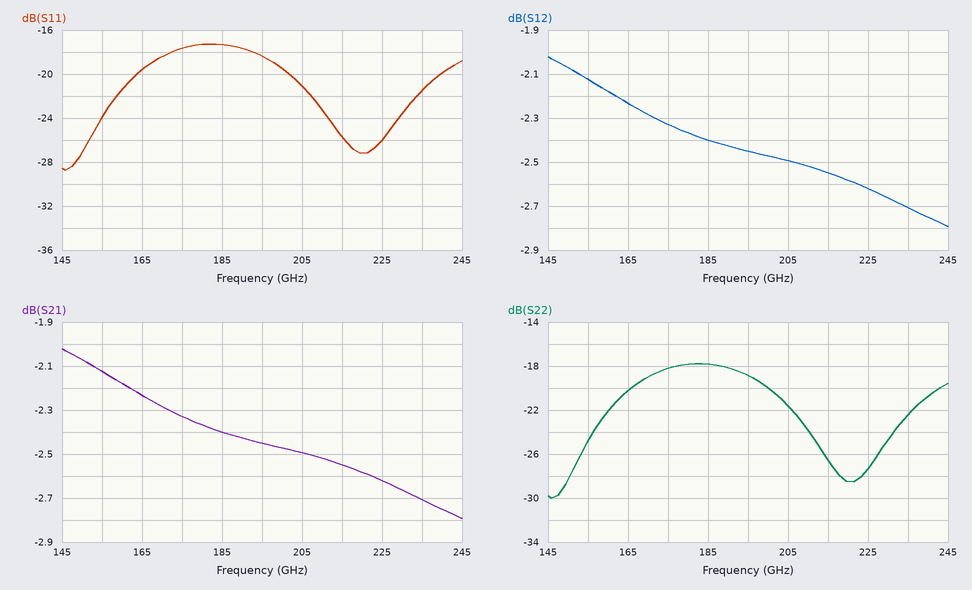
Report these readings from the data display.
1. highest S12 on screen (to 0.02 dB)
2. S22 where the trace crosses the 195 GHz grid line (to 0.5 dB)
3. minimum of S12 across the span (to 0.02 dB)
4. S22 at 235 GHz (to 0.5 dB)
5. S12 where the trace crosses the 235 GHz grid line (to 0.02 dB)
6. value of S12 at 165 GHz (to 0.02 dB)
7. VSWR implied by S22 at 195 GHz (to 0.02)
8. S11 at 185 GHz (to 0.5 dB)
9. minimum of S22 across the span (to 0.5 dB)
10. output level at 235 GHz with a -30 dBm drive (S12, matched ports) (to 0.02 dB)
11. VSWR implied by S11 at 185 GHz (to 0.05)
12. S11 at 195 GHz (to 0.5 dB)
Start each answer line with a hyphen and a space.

- -2.02 dB
- -19.0 dB
- -2.80 dB
- -22.5 dB
- -2.70 dB
- -2.24 dB
- 1.26
- -17.5 dB
- -30.0 dB
- -32.70 dBm
- 1.30
- -18.5 dB
